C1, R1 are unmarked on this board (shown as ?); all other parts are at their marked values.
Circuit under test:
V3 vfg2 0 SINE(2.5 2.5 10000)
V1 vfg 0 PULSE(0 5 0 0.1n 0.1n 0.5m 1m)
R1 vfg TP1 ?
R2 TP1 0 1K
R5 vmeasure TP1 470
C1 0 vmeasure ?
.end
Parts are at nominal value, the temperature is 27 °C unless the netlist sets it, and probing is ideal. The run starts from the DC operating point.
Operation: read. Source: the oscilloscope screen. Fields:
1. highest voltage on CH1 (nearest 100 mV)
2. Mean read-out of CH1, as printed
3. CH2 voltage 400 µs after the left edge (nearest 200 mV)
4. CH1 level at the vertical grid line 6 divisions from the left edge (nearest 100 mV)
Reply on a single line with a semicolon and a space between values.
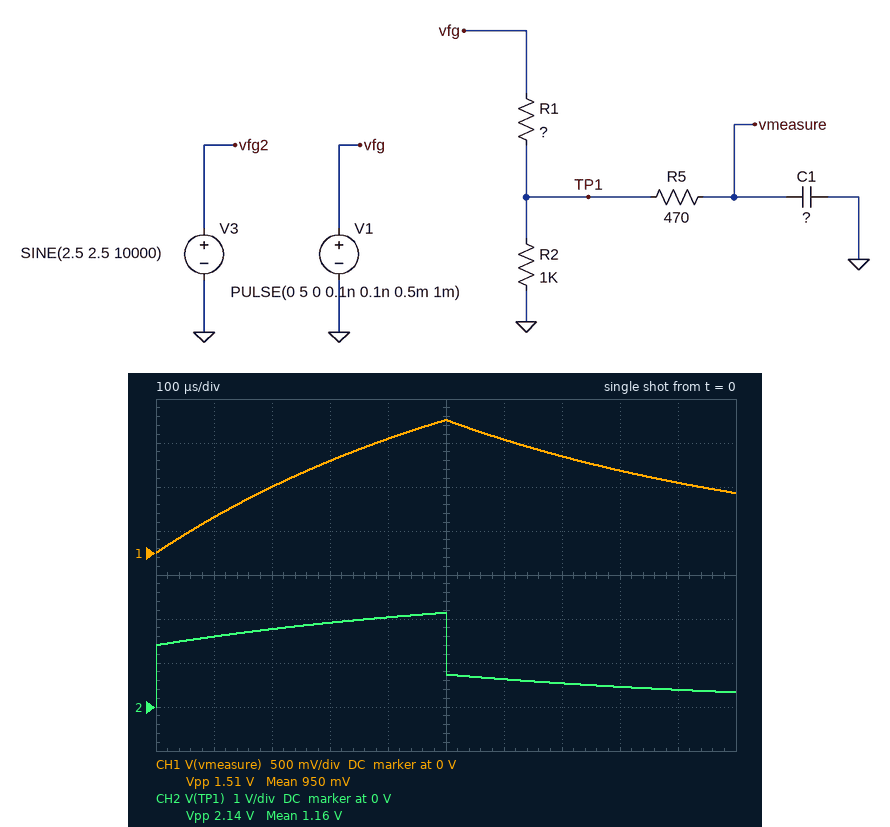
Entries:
1.5 V; 950 mV; 2.0 V; 1.3 V
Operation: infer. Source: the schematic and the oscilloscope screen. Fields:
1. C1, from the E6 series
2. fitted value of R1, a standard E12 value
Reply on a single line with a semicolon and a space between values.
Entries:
680 nF; 820 Ω
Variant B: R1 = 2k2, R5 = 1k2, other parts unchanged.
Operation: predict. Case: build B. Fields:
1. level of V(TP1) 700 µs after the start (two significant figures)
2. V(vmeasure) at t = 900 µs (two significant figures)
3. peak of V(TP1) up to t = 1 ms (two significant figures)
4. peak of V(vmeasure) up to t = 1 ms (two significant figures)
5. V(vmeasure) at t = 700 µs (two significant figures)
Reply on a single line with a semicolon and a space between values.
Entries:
160 mV; 370 mV; 1.2 V; 500 mV; 430 mV
